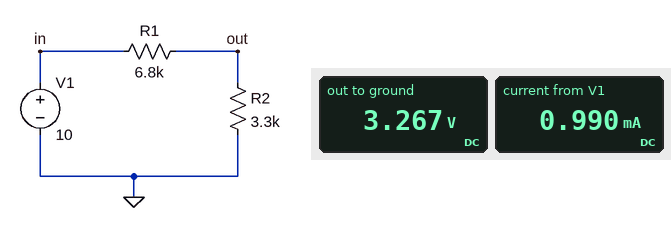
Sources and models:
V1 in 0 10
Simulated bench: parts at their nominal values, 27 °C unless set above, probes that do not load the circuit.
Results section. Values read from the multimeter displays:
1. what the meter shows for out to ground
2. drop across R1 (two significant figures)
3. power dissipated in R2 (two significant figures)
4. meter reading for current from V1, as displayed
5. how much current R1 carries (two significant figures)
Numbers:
3.267 V
6.7 V
3.2 mW
0.990 mA
990 µA
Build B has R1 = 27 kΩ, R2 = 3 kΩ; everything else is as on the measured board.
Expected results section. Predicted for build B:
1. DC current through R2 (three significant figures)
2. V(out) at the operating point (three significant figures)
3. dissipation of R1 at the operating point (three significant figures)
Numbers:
333 µA
1.00 V
3.00 mW
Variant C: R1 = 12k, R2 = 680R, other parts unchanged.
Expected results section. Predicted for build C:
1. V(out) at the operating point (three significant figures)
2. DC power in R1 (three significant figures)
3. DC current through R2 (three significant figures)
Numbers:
536 mV
7.46 mW
789 µA
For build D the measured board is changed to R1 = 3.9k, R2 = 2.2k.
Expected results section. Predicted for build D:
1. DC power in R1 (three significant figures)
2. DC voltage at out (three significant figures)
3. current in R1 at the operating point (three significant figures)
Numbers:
10.5 mW
3.61 V
1.64 mA
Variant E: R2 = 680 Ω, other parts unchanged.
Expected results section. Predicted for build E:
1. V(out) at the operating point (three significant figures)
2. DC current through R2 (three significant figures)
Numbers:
909 mV
1.34 mA
